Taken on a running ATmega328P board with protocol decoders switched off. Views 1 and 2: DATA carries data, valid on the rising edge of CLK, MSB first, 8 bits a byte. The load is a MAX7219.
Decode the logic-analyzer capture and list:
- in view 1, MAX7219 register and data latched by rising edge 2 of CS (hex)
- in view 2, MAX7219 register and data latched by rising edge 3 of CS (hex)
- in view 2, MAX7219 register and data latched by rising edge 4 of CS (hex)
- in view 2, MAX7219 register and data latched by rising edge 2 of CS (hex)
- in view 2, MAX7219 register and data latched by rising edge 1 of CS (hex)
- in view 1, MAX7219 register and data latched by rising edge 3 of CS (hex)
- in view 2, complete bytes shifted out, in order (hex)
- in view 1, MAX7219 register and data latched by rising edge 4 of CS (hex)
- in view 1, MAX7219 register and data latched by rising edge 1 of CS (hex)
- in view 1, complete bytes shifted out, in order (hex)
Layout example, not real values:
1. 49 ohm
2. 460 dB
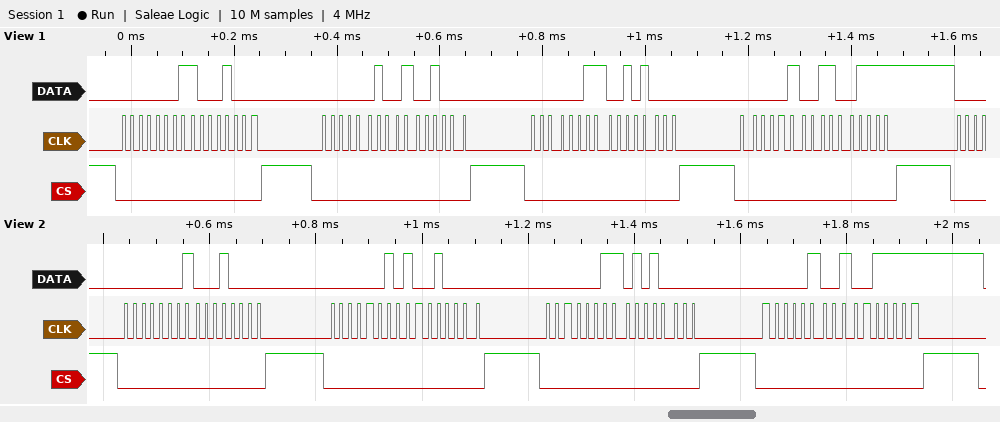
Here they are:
1. register 0x2, data 0x48
2. register 0x3, data 0x50
3. register 0x4, data 0x9F
4. register 0x2, data 0x90
5. register 0x1, data 0x10
6. register 0x3, data 0x28
7. 01 10 02 90 03 50 04 9F
8. register 0x4, data 0xCF
9. register 0x1, data 0x88
10. 0x01 0x88 0x02 0x48 0x03 0x28 0x04 0xCF
